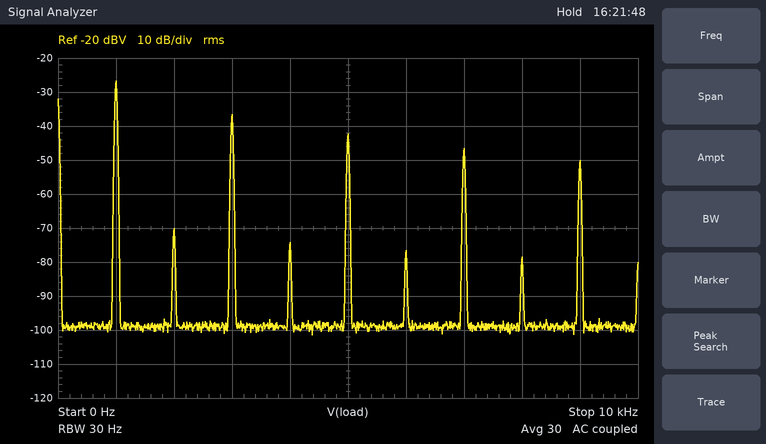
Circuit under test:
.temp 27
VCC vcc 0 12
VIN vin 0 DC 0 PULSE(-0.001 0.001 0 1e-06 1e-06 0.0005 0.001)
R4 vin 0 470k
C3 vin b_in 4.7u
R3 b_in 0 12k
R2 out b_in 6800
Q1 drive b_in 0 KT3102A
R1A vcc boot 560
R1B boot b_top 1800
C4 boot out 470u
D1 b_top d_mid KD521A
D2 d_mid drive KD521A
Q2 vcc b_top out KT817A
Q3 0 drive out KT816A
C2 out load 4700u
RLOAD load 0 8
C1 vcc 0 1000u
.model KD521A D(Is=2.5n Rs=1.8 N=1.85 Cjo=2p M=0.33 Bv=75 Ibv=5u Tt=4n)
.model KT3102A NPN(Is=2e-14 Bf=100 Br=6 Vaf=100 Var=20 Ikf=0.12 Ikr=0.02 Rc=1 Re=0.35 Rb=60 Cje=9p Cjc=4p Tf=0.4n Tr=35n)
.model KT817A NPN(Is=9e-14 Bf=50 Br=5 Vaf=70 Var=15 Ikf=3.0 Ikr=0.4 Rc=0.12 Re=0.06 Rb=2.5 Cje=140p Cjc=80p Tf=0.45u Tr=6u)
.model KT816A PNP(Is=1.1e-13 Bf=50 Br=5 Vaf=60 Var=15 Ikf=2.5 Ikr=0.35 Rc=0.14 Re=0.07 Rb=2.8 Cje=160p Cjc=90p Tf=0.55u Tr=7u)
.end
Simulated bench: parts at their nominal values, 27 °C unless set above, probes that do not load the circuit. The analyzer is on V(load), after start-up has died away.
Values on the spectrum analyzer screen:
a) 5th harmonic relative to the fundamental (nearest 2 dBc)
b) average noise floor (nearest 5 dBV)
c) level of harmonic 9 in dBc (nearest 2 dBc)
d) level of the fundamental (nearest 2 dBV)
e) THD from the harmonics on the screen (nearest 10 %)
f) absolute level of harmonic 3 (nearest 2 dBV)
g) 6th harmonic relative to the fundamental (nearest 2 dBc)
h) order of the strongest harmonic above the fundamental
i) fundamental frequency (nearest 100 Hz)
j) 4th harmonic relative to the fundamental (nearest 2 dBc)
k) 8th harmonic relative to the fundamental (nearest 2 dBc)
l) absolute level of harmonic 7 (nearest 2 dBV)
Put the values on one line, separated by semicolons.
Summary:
-16 dBc; -100 dBV; -24 dBc; -26 dBV; 40 %; -36 dBV; -50 dBc; 3; 1.0 kHz; -48 dBc; -52 dBc; -46 dBV
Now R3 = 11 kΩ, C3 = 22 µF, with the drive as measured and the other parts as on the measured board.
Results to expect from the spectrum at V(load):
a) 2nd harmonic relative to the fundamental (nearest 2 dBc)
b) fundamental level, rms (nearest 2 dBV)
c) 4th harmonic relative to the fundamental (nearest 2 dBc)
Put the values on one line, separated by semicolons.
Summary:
-48 dBc; -26 dBV; -50 dBc
